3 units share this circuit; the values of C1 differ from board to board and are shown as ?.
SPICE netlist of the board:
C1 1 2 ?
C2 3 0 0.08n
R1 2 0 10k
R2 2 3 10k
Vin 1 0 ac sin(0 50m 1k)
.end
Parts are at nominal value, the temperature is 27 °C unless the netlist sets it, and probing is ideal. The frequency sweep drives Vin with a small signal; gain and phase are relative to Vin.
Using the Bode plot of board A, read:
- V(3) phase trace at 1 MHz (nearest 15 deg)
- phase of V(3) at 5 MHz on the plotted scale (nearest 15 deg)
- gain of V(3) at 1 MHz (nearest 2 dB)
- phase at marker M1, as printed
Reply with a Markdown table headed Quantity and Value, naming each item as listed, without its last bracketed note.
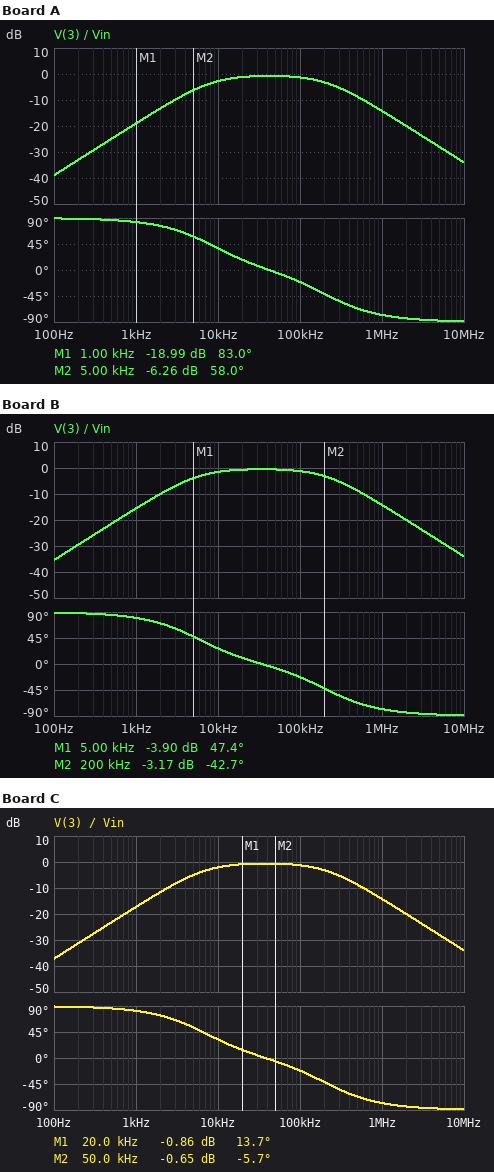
| Quantity | Value |
|---|---|
| V(3) phase trace at 1 MHz | -75 deg |
| phase of V(3) at 5 MHz on the plotted scale | -90 deg |
| gain of V(3) at 1 MHz | -14 dB |
| phase at marker M1, as printed | 83.0 deg |
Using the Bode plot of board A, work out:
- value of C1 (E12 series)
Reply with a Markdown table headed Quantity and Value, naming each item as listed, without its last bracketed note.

| Quantity | Value |
|---|---|
| value of C1 | 1.8 nF |
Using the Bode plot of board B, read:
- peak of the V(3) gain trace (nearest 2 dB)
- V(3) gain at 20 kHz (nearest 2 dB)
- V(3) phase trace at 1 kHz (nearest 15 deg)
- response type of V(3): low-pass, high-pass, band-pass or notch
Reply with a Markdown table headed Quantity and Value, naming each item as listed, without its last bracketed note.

| Quantity | Value |
|---|---|
| peak of the V(3) gain trace | 0 dB |
| V(3) gain at 20 kHz | 0 dB |
| V(3) phase trace at 1 kHz | 75 deg |
| response type of V(3): low-pass, high-pass, band-pass or notch | band-pass |
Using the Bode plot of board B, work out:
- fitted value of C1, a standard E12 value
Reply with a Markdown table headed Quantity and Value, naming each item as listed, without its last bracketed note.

| Quantity | Value |
|---|---|
| fitted value of C1, a standard E12 value | 2.7 nF |
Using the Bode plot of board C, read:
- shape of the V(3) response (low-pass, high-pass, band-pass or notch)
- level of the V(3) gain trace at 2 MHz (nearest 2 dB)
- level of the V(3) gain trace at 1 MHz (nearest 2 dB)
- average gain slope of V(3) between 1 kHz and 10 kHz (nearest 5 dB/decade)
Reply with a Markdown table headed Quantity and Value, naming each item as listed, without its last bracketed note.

| Quantity | Value |
|---|---|
| shape of the V(3) response | band-pass |
| level of the V(3) gain trace at 2 MHz | -20 dB |
| level of the V(3) gain trace at 1 MHz | -14 dB |
| average gain slope of V(3) between 1 kHz and 10 kHz | 15 dB/decade |
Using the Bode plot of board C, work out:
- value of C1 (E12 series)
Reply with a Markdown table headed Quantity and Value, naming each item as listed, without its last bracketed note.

| Quantity | Value |
|---|---|
| value of C1 | 2.2 nF |
